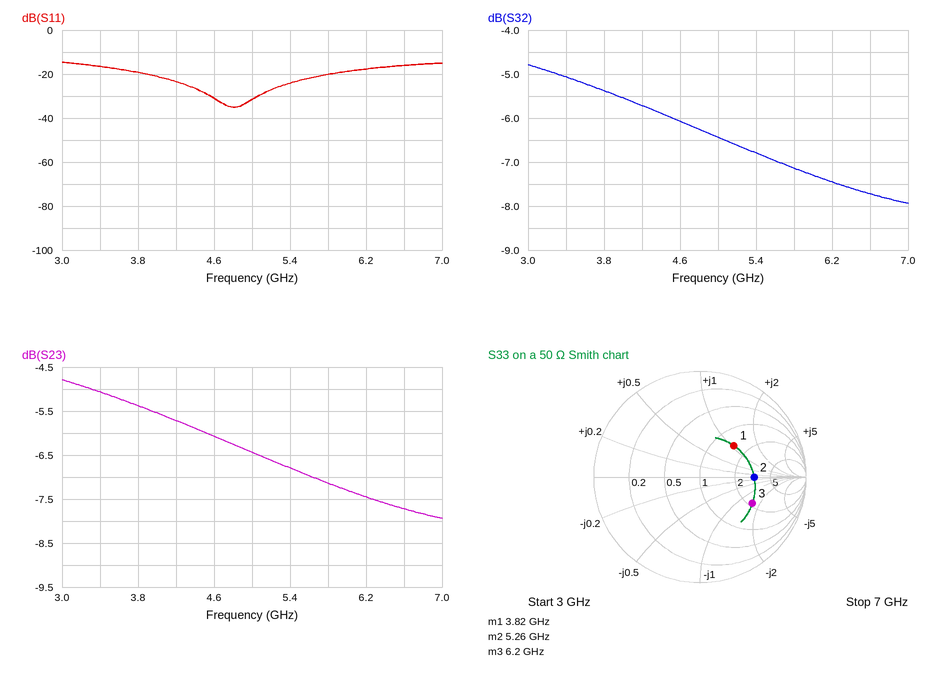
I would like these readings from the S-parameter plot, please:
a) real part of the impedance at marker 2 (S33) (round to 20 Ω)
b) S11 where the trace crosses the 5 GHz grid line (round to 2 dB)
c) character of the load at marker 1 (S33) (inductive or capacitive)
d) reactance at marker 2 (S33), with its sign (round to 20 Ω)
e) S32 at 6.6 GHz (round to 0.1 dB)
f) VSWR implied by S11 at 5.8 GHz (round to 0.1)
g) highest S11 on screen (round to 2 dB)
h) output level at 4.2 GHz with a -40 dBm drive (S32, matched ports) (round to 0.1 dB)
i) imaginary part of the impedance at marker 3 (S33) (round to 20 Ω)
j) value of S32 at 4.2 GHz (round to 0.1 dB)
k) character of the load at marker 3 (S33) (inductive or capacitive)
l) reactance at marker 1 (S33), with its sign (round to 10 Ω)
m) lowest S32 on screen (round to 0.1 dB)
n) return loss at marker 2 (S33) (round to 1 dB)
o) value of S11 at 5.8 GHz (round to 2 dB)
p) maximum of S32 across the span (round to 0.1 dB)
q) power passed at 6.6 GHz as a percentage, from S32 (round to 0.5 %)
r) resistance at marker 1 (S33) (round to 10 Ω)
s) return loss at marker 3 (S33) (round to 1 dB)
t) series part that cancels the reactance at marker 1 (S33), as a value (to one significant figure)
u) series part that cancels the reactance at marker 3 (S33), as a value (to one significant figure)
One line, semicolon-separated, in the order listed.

160 Ω; -32 dB; inductive; 0 Ω; -7.7 dB; 1.2; -14 dB; -45.7 dBm; -80 Ω; -5.7 dB; capacitive; +50 Ω; -7.9 dB; 6 dB; -20 dB; -4.8 dB; 17.0 %; 70 Ω; 5 dB; 800 fF; 2 nH
